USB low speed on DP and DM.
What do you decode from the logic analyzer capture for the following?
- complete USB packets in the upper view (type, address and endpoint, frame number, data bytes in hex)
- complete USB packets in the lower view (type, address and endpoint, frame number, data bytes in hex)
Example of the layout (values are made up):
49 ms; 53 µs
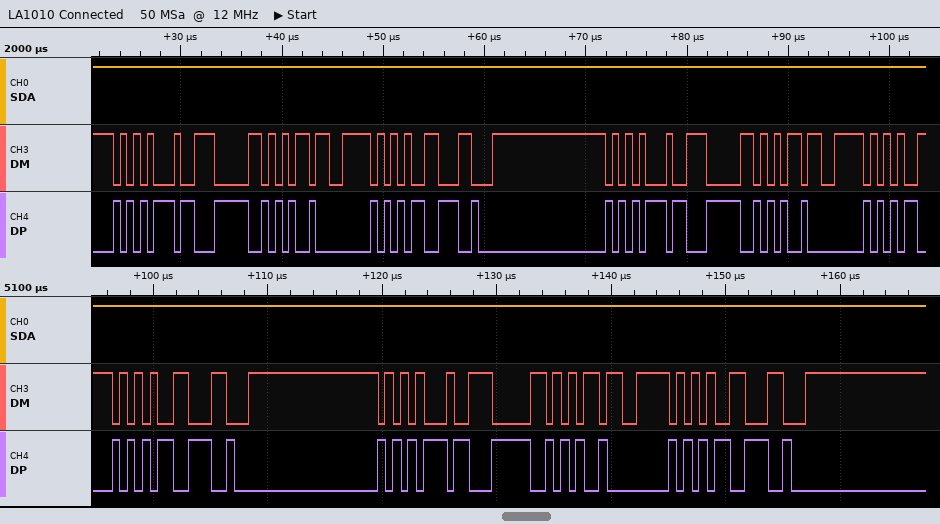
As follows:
IN ADDR 47 EP 0, NAK, IN ADDR 47 EP 0; NAK, IN ADDR 47 EP 0, NAK
